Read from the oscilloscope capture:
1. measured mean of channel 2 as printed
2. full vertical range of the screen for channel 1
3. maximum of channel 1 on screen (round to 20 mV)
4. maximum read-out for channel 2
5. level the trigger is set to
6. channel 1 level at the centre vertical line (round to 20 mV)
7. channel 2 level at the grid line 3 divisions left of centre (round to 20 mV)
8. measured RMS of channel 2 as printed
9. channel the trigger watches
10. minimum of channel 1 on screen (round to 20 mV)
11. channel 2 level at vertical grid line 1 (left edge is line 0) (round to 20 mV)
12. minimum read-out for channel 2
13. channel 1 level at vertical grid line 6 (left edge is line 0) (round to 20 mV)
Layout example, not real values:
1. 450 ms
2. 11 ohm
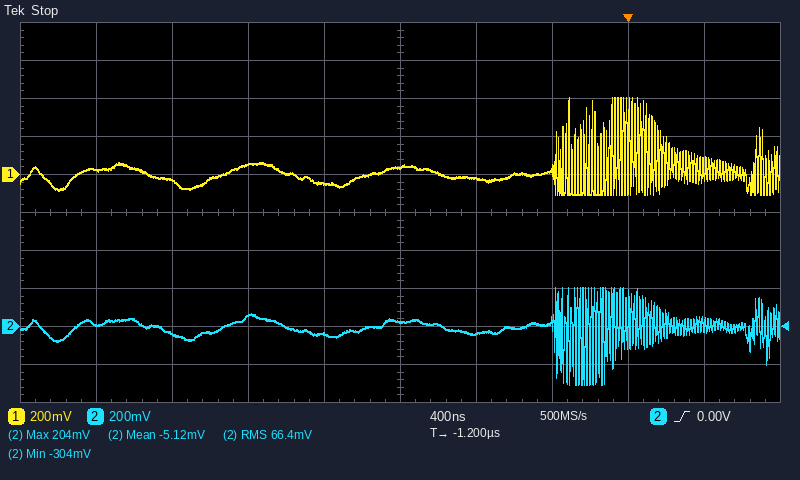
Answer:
1. -5.12 mV
2. 2 V
3. 400 mV
4. 204 mV
5. 0.00 V
6. 40 mV
7. -40 mV
8. 66.4 mV
9. channel 2
10. -100 mV
11. 20 mV
12. -304 mV
13. -20 mV
